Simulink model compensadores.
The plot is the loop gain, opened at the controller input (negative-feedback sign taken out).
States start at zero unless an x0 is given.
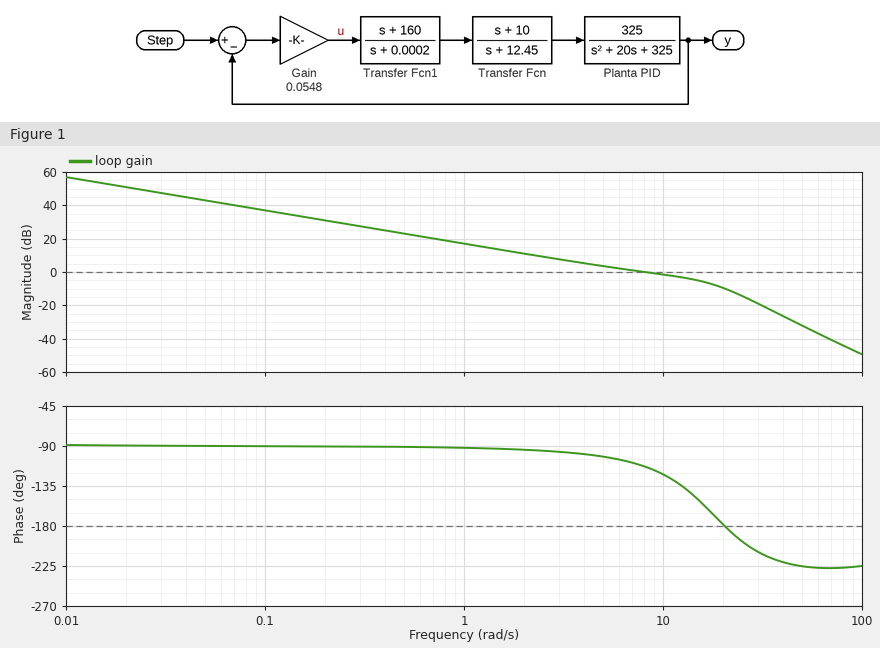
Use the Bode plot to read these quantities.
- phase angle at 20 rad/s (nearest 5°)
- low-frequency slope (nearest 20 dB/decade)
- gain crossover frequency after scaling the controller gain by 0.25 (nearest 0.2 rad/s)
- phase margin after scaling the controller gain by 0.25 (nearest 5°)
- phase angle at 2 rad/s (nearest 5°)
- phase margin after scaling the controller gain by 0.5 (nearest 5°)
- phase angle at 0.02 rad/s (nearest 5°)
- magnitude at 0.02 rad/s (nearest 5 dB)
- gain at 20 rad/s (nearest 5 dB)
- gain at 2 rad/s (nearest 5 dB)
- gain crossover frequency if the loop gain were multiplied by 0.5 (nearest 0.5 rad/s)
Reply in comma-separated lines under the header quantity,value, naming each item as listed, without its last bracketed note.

quantity,value
phase angle at 20 rad/s,-180°
low-frequency slope,-20 dB/decade
gain crossover frequency after scaling the controller gain by 0.25,1.8 rad/s
phase margin after scaling the controller gain by 0.25,85°
phase angle at 2 rad/s,-95°
phase margin after scaling the controller gain by 0.5,80°
phase angle at 0.02 rad/s,-90°
magnitude at 0.02 rad/s,50 dB
gain at 20 rad/s,-10 dB
gain at 2 rad/s,10 dB
gain crossover frequency if the loop gain were multiplied by 0.5,3.5 rad/s
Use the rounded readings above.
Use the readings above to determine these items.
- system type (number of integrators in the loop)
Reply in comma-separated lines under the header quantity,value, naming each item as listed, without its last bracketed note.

quantity,value
system type,1
